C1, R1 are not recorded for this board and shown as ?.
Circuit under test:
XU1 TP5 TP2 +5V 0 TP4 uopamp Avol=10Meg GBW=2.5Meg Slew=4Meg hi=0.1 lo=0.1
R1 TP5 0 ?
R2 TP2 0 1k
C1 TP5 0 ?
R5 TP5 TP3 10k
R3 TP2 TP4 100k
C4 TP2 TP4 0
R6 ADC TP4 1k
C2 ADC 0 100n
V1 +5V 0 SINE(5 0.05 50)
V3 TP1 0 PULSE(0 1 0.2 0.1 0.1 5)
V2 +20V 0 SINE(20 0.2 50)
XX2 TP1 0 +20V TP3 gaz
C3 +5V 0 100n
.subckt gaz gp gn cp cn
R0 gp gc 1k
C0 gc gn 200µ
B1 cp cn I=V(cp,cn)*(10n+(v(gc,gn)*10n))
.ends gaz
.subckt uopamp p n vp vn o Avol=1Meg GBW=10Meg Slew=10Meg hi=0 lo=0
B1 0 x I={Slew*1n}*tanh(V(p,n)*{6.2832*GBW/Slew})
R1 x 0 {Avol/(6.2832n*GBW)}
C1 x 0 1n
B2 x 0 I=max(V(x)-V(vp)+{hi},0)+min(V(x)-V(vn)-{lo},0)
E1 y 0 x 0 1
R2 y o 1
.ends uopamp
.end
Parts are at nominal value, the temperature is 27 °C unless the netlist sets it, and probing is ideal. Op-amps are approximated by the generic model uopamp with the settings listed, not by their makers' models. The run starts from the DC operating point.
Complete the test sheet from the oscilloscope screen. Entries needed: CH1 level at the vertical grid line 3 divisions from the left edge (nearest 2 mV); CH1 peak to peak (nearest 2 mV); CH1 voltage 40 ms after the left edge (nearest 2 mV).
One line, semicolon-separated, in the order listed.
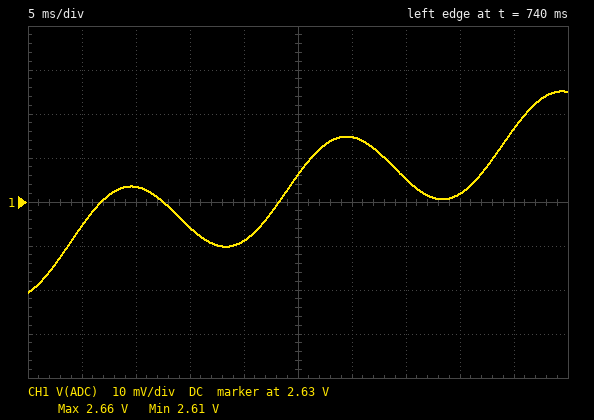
2.624 V; 46 mV; 2.632 V
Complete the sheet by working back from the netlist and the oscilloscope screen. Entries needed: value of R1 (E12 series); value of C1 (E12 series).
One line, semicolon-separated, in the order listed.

68 kΩ; 120 nF
